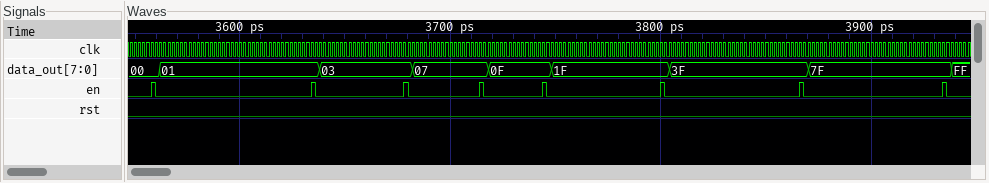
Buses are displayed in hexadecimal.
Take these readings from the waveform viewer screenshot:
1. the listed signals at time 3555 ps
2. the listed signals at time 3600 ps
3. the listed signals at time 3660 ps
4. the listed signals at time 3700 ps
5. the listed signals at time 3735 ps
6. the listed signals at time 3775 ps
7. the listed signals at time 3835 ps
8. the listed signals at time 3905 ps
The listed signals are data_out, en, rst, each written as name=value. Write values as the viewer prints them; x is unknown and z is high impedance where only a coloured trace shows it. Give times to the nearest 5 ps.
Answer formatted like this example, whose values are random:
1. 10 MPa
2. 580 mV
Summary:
1. data_out=00, en=0, rst=0
2. data_out=01, en=0, rst=0
3. data_out=03, en=0, rst=0
4. data_out=07, en=0, rst=0
5. data_out=0F, en=0, rst=0
6. data_out=1F, en=0, rst=0
7. data_out=3F, en=0, rst=0
8. data_out=7F, en=0, rst=0
